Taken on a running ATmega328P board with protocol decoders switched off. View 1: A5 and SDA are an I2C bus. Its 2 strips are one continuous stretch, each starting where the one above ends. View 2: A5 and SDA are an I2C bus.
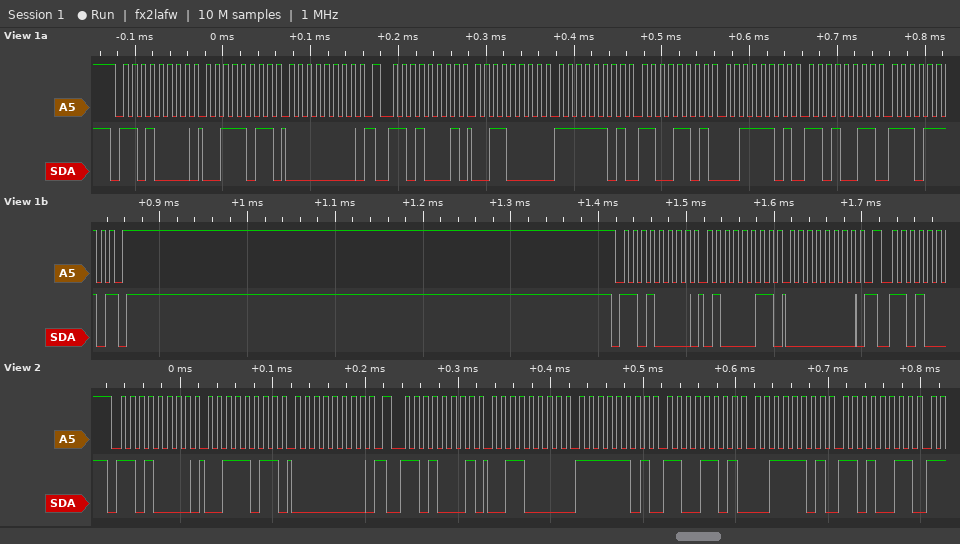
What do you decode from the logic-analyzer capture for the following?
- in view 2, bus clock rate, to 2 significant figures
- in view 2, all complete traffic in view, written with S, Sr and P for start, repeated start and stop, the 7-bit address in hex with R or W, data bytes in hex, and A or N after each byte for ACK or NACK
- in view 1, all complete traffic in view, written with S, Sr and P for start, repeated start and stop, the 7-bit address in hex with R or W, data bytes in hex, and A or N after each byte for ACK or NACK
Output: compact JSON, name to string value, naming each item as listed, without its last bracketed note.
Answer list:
{"in view 2, bus clock rate, to 2 significant figures": "100 kHz", "in view 2, all complete traffic in view, written with S, Sr and P for start, repeated start and stop, the 7-bit address in hex with R or W, data bytes in hex, and A or N after each byte for ACK or NACK": "S 68W A 3B A 00 A Sr 68R A 30 A FD A CD A 3D A D3 A", "in view 1, all complete traffic in view, written with S, Sr and P for start, repeated start and stop, the 7-bit address in hex with R or W, data bytes in hex, and A or N after each byte for ACK or NACK": "S 68W A 3B A 00 A Sr 68R A 30 A FD A CD A 3D A D3 A EE N P S 68W A 43 A 00 A"}
